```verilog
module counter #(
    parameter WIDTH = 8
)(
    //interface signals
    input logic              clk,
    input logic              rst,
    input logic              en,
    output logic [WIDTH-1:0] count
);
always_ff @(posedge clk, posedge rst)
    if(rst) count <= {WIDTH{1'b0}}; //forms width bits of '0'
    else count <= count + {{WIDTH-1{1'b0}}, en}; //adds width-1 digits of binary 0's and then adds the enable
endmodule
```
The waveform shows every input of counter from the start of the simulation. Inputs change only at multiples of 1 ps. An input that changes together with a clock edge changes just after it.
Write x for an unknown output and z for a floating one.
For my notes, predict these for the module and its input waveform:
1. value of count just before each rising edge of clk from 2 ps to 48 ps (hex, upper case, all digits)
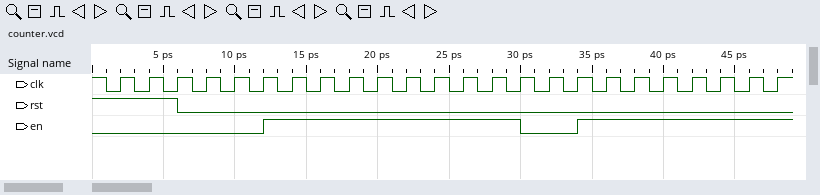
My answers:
00, 00, 00, 00, 00, 00, 00, 01, 02, 03, 04, 05, 06, 07, 08, 09, 09, 09, 0A, 0B, 0C, 0D, 0E, 0F
